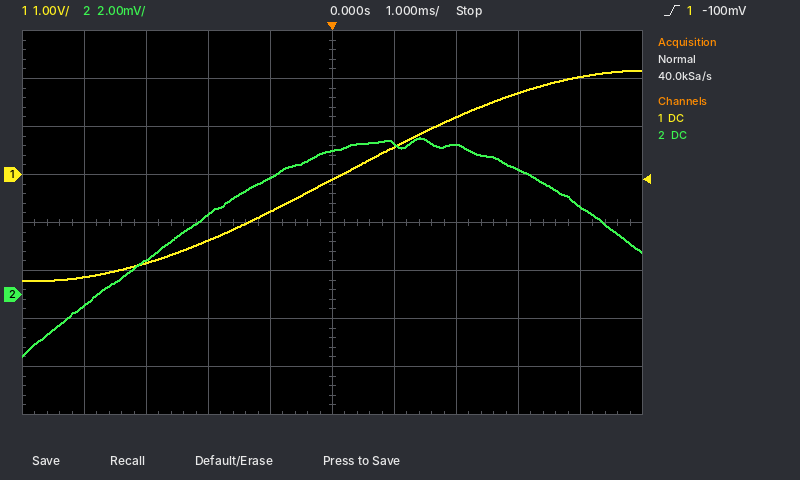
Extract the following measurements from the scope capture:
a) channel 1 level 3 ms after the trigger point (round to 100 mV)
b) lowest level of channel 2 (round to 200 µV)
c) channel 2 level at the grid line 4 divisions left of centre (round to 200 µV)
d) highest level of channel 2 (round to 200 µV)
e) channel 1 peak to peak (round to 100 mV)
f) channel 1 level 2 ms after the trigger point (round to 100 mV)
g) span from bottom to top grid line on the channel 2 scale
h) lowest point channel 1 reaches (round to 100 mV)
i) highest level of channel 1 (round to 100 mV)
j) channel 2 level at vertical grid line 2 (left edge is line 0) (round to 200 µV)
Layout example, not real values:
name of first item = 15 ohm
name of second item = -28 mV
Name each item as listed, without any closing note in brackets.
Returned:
channel 1 level 3 ms after the trigger point = 1.7 V
lowest level of channel 2 = -2.6 mV
channel 2 level at the grid line 4 divisions left of centre = -400 µV
highest level of channel 2 = 6.6 mV
channel 1 peak to peak = 4.4 V
channel 1 level 2 ms after the trigger point = 1.2 V
span from bottom to top grid line on the channel 2 scale = 16 mV
lowest point channel 1 reaches = -2.2 V
highest level of channel 1 = 2.2 V
channel 2 level at vertical grid line 2 (left edge is line 0) = 1.4 mV
